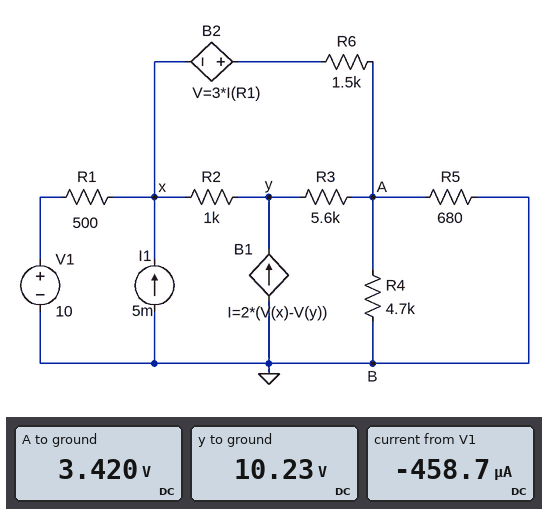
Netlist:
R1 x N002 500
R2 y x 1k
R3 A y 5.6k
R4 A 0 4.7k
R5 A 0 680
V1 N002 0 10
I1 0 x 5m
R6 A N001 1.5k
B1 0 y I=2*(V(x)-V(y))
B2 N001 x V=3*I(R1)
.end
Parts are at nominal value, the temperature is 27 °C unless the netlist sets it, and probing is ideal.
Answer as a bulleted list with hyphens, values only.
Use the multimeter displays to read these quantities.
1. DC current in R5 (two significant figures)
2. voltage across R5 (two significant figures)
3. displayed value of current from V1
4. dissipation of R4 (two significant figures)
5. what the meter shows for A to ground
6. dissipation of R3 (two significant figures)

- 5.0 mA
- 3.4 V
- -458.7 µA
- 2.5 mW
- 3.420 V
- 8.3 mW
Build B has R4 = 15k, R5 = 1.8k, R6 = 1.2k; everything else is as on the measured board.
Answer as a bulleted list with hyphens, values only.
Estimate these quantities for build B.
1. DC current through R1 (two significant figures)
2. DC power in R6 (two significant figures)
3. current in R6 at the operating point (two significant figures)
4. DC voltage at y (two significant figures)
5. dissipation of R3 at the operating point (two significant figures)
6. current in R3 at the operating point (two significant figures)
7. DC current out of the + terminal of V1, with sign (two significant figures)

- 1.6 mA
- 14 mW
- 3.4 mA
- 11 V
- 3.0 mW
- 730 µA
- -1.6 mA
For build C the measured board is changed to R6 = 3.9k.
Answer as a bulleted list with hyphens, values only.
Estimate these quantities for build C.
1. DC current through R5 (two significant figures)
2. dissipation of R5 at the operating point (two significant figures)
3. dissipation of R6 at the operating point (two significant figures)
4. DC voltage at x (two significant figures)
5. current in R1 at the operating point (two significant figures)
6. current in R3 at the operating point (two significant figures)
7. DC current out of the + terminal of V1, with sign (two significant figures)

- 3.4 mA
- 8.0 mW
- 21 mW
- 11 V
- 2.7 mA
- 1.6 mA
- -2.7 mA
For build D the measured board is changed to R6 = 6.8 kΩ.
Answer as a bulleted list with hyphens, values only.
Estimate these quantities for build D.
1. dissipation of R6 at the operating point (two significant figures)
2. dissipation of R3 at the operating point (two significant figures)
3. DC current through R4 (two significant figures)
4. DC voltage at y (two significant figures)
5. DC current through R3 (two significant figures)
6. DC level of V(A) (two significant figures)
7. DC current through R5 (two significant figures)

- 14 mW
- 17 mW
- 410 µA
- 12 V
- 1.8 mA
- 1.9 V
- 2.8 mA
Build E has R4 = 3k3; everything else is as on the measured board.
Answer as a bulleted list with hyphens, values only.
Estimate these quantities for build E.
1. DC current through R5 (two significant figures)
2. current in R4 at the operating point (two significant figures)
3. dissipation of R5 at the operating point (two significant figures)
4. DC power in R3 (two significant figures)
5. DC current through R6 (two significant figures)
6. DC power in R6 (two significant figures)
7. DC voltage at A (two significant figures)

- 4.8 mA
- 1.0 mA
- 16 mW
- 8.5 mW
- 4.6 mA
- 32 mW
- 3.3 V
